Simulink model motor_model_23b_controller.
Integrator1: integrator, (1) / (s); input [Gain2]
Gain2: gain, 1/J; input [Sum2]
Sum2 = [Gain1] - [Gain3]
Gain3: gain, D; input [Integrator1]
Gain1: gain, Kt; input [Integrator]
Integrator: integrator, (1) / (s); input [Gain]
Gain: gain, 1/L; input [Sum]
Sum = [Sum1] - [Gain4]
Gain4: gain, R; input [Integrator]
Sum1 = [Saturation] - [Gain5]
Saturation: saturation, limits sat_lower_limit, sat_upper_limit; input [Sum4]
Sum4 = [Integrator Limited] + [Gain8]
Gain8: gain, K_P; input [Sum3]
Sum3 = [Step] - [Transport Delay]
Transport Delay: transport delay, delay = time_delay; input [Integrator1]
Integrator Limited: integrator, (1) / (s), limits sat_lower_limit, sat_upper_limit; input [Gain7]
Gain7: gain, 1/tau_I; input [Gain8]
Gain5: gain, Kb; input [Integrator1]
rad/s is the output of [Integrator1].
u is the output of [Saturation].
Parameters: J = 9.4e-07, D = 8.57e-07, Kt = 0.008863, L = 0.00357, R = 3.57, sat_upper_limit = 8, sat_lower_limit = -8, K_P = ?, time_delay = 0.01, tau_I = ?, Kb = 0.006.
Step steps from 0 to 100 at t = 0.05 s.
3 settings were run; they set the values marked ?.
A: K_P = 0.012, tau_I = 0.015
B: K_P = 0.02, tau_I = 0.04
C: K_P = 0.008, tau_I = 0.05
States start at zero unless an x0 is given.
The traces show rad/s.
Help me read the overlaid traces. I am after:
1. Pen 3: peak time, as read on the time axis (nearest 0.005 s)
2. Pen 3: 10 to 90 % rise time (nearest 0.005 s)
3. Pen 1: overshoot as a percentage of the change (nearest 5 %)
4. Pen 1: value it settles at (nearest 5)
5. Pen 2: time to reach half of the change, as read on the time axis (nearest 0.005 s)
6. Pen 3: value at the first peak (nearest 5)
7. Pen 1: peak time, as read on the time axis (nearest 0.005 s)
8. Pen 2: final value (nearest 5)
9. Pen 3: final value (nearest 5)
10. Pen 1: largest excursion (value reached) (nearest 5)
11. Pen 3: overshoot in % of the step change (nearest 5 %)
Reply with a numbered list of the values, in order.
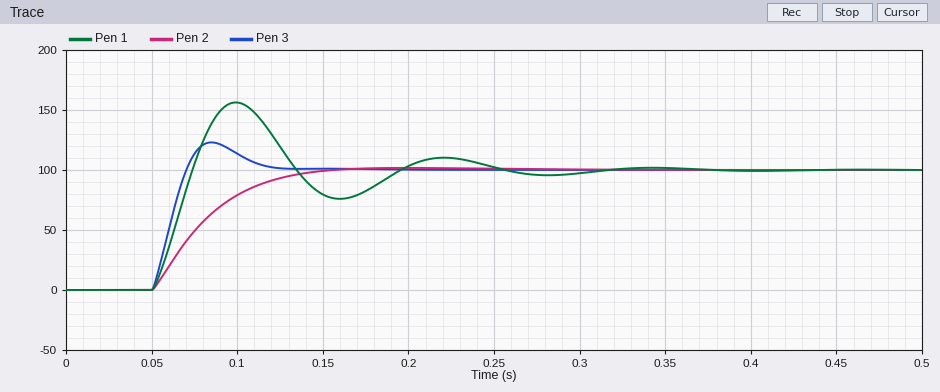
1. 0.085 s
2. 0.015 s
3. 55 %
4. 100
5. 0.075 s
6. 125
7. 0.100 s
8. 100
9. 100
10. 155
11. 25 %
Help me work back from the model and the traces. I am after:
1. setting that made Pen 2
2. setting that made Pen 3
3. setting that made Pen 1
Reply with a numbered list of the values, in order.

1. C
2. B
3. A
